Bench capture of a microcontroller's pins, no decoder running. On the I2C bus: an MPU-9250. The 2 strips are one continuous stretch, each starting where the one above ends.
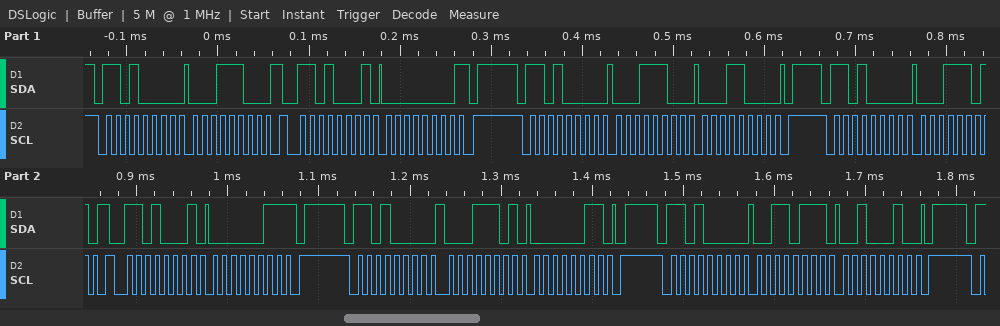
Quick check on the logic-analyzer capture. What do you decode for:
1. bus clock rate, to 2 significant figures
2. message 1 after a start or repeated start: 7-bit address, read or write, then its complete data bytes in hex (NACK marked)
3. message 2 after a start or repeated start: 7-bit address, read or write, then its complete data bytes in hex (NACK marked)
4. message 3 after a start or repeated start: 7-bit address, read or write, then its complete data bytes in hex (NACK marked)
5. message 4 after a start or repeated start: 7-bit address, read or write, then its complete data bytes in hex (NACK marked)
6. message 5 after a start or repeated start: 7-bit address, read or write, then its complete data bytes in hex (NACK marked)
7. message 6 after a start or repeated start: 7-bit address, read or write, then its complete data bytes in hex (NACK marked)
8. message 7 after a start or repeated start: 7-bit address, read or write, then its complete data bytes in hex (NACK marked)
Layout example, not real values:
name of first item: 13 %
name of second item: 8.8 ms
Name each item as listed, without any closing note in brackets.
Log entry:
bus clock rate, to 2 significant figures: 100 kHz
message 1 after a start or repeated start: 7-bit address, read or write, then its complete data bytes in hex: 0x68 write: 1C
message 2 after a start or repeated start: 7-bit address, read or write, then its complete data bytes in hex: 0x68 read: 00 NACK
message 3 after a start or repeated start: 7-bit address, read or write, then its complete data bytes in hex: 0x68 write: 1C 18
message 4 after a start or repeated start: 7-bit address, read or write, then its complete data bytes in hex: 0x68 write: 1D
message 5 after a start or repeated start: 7-bit address, read or write, then its complete data bytes in hex: 0x68 read: 03 NACK
message 6 after a start or repeated start: 7-bit address, read or write, then its complete data bytes in hex: 0x68 write: 1D 03
message 7 after a start or repeated start: 7-bit address, read or write, then its complete data bytes in hex: 0x68 write: 37 22
